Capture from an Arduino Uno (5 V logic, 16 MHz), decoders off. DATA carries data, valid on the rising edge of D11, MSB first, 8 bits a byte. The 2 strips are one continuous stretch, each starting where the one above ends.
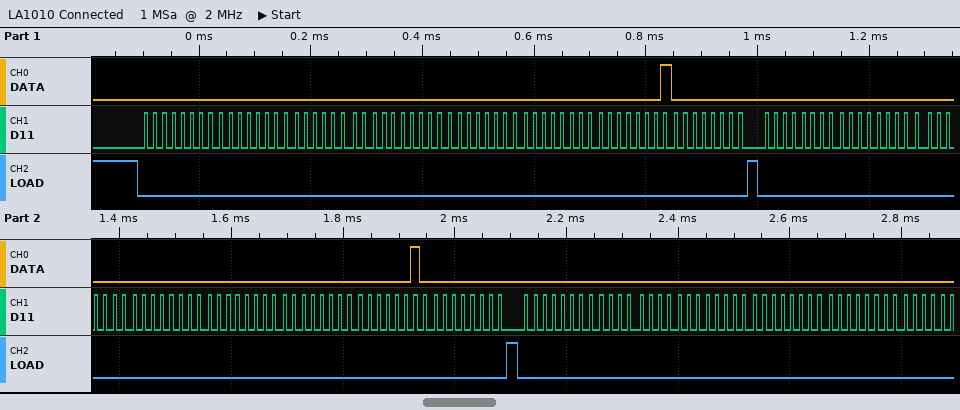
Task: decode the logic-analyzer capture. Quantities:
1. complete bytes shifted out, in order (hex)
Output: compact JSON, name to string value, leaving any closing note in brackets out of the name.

{"complete bytes shifted out, in order": "0x00 0x00 0x00 0x00 0x00 0x00 0x01 0x00 0x00 0x00 0x00 0x00 0x00 0x00 0x02 0x00 0x00 0x00 0x00 0x00 0x00"}
